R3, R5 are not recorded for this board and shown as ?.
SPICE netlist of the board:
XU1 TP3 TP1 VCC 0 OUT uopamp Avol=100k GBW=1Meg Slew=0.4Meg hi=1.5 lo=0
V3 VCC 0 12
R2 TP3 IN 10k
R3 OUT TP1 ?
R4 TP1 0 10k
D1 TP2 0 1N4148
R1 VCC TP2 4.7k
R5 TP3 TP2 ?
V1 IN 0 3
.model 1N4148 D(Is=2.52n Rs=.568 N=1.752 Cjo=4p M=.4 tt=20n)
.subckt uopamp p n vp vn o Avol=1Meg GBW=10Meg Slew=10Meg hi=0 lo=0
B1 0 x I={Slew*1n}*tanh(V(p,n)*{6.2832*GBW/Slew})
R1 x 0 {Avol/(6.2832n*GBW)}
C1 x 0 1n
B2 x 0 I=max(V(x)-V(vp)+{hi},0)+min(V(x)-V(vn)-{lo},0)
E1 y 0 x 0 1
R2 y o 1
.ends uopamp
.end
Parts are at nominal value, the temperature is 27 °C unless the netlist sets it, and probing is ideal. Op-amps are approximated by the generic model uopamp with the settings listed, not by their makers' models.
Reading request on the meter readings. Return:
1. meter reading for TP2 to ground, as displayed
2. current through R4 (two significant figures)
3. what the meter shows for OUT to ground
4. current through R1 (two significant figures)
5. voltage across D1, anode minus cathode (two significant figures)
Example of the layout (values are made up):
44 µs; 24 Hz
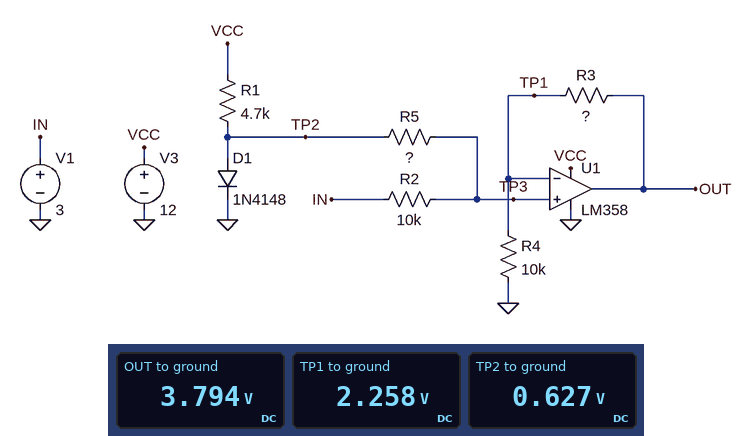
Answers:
0.627 V; 230 µA; 3.794 V; 2.4 mA; 630 mV
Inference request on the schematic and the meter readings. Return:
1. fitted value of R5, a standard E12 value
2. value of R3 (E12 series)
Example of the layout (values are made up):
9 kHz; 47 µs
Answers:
22 kΩ; 6.8 kΩ
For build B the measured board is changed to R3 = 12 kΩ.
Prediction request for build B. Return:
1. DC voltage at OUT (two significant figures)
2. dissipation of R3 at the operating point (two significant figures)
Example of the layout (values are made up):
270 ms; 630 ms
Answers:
5.0 V; 610 µW
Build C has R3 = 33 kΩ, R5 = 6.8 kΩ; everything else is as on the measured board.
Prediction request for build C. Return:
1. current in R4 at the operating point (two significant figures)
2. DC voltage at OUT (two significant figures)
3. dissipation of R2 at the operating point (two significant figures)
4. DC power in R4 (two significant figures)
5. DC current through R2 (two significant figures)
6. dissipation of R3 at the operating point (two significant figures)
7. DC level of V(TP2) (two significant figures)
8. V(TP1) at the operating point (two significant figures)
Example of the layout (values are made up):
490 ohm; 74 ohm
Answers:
160 µA; 6.8 V; 200 µW; 250 µW; 140 µA; 830 µW; 630 mV; 1.6 V
